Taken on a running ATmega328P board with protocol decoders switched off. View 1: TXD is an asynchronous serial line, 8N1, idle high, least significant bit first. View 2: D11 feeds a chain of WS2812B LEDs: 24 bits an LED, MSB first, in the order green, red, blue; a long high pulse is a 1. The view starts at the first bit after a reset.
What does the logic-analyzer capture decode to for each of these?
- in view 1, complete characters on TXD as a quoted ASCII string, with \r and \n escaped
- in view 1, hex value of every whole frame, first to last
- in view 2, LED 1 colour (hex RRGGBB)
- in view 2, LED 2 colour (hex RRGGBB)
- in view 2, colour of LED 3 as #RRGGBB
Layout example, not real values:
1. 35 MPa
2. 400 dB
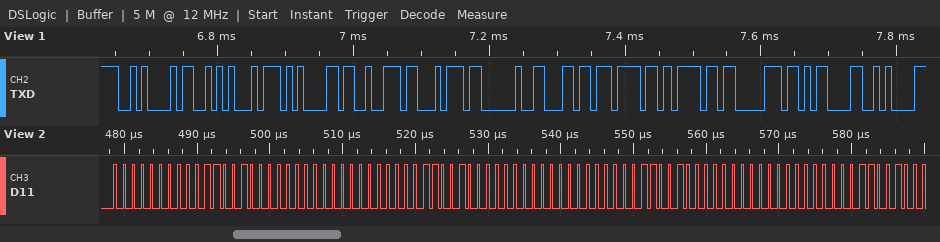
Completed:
1. "\nStart loop\r\n"
2. 0A 53 74 61 72 74 20 6C 6F 6F 70 0D 0A
3. #320000
4. #320000
5. #320000
